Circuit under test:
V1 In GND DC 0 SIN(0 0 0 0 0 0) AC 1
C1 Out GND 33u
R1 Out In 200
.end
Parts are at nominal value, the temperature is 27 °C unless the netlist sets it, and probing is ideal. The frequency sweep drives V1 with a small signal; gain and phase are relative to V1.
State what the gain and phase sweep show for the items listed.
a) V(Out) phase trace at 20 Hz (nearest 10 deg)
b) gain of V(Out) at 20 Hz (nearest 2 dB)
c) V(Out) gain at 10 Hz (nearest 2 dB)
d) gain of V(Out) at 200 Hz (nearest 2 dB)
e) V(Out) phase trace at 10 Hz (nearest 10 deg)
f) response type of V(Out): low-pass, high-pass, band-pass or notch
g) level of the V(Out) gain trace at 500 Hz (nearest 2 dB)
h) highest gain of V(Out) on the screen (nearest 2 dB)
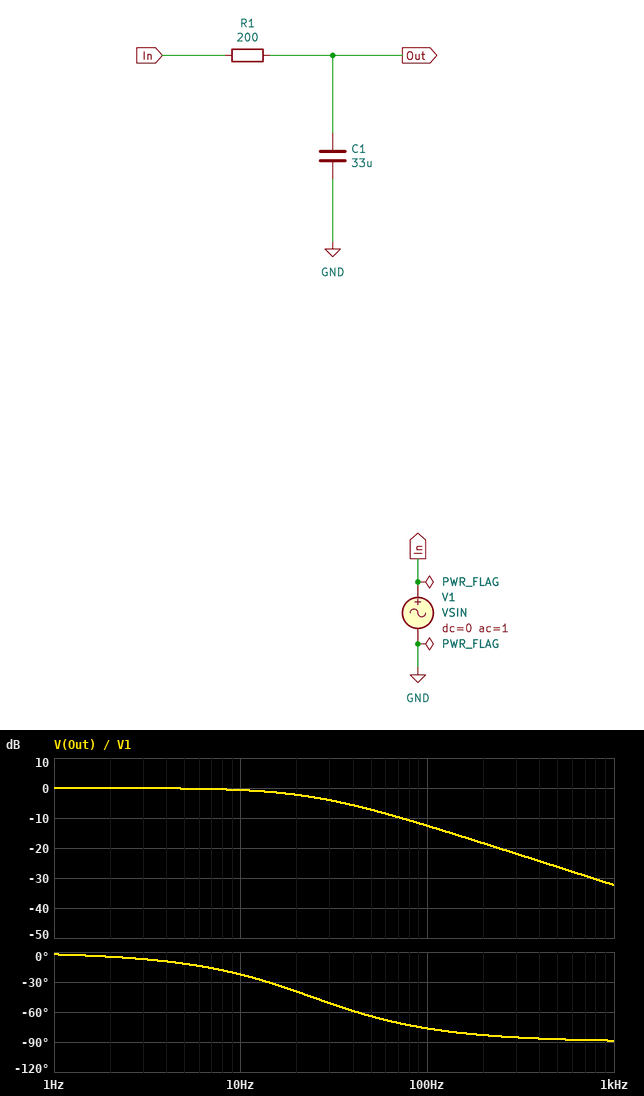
-40 deg
-2 dB
0 dB
-18 dB
-20 deg
low-pass
-26 dB
0 dB
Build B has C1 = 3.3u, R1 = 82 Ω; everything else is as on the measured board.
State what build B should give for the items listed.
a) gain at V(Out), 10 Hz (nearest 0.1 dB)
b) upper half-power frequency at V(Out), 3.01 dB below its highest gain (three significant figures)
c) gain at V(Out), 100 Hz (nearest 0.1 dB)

0 dB
588 Hz
-0.1 dB
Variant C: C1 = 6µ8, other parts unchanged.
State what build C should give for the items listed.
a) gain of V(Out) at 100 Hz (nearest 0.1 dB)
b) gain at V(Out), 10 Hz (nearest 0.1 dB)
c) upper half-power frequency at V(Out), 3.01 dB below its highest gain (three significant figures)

-2.4 dB
0 dB
117 Hz
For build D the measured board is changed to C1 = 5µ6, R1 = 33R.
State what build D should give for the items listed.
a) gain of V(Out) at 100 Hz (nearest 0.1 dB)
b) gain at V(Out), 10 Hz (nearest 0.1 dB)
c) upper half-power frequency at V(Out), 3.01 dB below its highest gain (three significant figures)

-0.1 dB
0 dB
861 Hz
